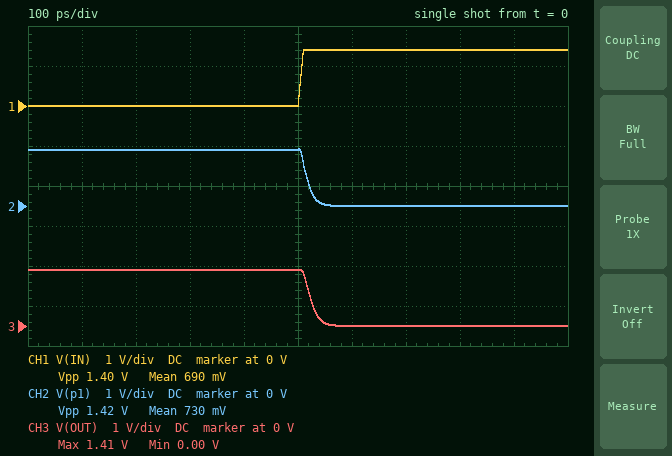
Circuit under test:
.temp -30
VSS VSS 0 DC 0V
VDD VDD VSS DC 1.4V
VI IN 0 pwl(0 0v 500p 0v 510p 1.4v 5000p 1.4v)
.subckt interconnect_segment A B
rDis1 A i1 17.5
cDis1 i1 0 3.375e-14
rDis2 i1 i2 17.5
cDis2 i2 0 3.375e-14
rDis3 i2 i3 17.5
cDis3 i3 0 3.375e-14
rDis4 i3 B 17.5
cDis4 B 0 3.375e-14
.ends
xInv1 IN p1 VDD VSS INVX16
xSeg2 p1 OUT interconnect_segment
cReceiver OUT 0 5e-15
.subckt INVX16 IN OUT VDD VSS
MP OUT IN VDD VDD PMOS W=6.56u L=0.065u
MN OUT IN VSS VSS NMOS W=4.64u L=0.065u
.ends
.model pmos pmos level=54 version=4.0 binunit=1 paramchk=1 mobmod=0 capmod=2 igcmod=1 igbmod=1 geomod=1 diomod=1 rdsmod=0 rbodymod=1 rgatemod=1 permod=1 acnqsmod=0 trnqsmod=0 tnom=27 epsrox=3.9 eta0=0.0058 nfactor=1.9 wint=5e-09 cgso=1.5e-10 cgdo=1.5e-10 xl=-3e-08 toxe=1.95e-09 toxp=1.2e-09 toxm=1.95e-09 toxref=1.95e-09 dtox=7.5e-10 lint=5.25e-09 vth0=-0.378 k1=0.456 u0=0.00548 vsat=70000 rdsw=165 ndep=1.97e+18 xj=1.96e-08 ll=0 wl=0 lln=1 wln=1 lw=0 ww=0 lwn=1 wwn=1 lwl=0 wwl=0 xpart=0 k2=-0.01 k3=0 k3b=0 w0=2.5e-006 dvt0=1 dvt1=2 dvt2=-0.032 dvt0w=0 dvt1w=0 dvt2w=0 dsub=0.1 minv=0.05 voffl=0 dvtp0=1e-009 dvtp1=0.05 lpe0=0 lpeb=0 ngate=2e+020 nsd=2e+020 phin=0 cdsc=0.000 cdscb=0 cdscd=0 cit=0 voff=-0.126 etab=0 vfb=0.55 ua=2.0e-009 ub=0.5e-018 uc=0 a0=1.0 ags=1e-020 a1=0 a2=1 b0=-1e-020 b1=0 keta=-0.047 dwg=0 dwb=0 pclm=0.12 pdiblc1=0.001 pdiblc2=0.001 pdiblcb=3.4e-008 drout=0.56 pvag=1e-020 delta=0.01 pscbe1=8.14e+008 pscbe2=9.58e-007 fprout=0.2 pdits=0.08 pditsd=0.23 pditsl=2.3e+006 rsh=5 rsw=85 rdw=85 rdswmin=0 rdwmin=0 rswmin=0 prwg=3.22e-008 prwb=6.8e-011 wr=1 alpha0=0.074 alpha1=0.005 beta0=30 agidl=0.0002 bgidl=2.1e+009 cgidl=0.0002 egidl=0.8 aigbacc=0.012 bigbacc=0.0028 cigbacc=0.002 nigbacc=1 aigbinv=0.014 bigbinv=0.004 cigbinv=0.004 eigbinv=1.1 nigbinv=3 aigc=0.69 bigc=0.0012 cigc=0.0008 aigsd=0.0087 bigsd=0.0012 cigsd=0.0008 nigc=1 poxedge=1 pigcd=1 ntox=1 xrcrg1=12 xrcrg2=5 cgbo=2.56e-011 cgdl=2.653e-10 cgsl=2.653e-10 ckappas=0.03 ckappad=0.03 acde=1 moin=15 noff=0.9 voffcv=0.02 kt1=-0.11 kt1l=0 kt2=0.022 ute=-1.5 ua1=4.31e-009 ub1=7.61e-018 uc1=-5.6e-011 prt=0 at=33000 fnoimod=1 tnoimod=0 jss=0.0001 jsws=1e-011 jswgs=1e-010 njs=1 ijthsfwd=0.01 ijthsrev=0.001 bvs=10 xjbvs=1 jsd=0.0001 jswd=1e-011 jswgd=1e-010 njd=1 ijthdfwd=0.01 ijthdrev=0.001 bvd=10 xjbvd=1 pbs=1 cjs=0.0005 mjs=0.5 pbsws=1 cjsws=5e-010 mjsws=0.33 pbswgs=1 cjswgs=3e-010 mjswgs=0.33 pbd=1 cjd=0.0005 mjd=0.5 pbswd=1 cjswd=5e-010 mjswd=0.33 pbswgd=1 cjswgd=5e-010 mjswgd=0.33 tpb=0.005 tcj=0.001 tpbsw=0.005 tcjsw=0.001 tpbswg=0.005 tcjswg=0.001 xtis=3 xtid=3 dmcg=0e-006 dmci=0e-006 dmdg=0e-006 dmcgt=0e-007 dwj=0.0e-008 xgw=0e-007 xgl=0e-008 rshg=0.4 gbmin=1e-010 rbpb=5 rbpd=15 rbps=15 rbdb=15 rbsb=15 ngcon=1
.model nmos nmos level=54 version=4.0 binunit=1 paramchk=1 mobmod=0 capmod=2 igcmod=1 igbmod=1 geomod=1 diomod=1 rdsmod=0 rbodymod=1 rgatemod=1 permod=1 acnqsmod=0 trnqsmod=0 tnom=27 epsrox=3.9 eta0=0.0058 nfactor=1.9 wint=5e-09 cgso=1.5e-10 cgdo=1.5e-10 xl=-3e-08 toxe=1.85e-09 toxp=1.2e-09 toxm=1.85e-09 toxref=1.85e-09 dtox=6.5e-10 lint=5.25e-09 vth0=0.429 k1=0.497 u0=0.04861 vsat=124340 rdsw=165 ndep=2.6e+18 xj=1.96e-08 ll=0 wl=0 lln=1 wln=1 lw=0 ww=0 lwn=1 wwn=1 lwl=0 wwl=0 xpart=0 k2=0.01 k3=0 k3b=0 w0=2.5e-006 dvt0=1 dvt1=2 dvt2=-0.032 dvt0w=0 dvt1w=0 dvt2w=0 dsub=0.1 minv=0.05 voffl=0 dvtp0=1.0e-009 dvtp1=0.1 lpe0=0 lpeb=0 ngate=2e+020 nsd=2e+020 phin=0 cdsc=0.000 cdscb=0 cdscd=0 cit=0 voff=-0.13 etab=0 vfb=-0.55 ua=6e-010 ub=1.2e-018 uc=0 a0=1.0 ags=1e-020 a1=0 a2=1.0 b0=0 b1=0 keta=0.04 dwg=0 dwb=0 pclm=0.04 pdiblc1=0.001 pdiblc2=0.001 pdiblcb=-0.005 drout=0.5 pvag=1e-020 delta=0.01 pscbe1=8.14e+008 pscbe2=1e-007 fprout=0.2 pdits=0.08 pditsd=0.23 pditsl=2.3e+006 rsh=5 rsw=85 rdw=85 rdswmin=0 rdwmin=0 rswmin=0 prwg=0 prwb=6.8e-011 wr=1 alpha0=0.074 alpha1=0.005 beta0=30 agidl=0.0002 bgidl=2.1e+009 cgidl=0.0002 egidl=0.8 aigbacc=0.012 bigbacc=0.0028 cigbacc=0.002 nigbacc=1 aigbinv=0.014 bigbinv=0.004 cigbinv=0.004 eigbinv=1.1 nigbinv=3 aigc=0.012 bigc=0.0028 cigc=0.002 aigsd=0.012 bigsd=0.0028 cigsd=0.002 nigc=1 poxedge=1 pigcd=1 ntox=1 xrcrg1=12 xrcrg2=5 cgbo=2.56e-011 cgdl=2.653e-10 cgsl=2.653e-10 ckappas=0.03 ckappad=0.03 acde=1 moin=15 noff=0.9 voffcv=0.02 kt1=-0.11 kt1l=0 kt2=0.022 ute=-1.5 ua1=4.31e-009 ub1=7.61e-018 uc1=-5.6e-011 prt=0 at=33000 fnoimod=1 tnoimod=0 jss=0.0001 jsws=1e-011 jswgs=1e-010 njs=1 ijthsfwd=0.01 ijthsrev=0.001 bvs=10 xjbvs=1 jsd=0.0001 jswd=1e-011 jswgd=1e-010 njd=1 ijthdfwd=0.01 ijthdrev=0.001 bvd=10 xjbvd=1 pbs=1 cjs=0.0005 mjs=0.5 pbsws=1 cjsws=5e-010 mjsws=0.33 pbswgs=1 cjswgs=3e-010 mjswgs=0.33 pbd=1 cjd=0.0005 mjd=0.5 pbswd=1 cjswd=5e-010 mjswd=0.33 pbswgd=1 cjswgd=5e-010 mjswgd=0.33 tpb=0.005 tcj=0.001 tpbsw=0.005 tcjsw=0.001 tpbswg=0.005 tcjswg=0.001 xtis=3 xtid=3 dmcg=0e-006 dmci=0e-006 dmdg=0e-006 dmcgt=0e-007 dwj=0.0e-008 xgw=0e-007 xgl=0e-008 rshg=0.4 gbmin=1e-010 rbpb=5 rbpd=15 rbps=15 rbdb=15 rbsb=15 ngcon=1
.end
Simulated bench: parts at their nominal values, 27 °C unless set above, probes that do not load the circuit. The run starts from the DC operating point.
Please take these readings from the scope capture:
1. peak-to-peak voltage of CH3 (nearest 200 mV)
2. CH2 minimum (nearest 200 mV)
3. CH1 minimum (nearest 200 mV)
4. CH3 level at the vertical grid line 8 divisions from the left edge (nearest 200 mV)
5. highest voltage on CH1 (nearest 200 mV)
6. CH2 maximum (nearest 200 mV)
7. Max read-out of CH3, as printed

1.4 V
0 V
0 V
0 V
1.4 V
1.4 V
1.41 V
